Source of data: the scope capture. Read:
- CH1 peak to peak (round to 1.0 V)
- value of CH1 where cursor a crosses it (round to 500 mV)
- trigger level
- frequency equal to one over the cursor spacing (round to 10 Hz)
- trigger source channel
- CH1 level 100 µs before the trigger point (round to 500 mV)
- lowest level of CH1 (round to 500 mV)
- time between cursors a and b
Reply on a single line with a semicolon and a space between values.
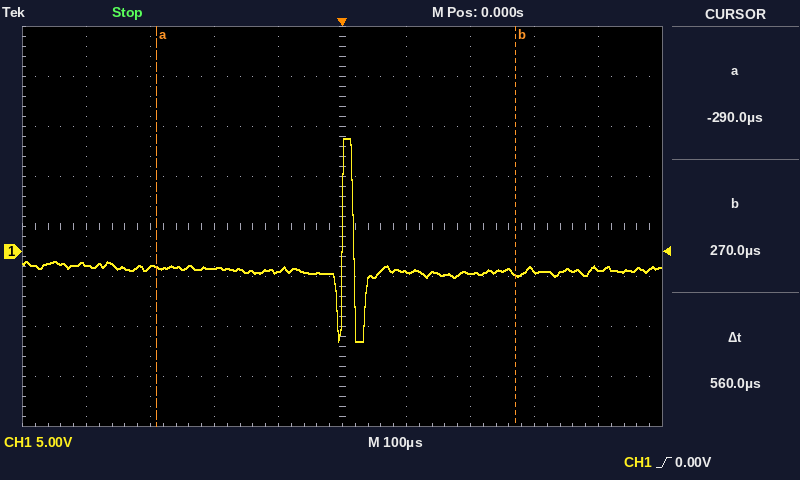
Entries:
20.0 V; -1.5 V; 0.00 V; 1.79 kHz; CH1; -2.0 V; -9.0 V; 560 µs
